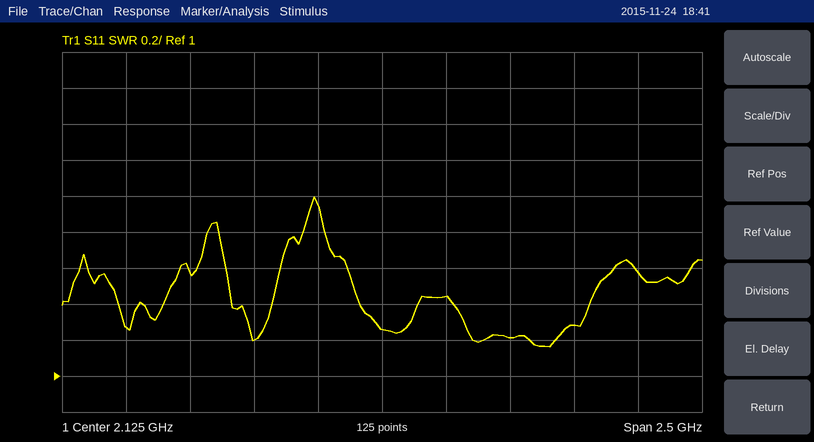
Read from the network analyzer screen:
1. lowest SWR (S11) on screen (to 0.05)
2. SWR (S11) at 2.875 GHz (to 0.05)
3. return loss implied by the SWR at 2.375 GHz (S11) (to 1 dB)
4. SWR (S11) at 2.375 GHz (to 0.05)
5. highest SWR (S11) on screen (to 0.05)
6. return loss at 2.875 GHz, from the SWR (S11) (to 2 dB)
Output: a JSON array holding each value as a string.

["1.15", "1.30", "15 dB", "1.45", "2.00", "18 dB"]
